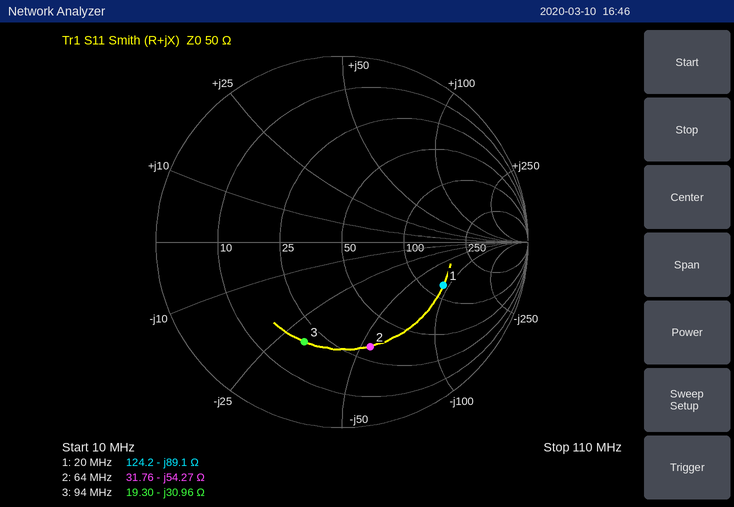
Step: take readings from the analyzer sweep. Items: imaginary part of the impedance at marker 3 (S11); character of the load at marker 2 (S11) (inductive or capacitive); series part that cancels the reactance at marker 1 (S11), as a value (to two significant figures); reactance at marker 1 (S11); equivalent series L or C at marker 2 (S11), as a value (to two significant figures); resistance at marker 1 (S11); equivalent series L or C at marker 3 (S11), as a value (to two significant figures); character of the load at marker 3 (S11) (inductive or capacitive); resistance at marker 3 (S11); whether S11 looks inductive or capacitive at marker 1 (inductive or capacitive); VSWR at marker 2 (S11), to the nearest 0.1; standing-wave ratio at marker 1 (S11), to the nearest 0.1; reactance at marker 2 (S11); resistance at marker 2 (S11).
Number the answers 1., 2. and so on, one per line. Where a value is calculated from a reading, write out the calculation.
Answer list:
1. -30.96 Ω
2. capacitive
3. L = 89.1 Ω/(2π × 20 MHz) ≈ 709 nH, so 710 nH to two significant figures
4. -89.1 Ω
5. C = 1/(2π × 64 MHz × 54.27 Ω) ≈ 46 pF
6. 124.2 Ω
7. C = 1/(2π × 94 MHz × 30.96 Ω) ≈ 55 pF
8. capacitive
9. 19.30 Ω
10. capacitive
11. 3.8
12. 3.9
13. -54.27 Ω
14. 31.76 Ω
